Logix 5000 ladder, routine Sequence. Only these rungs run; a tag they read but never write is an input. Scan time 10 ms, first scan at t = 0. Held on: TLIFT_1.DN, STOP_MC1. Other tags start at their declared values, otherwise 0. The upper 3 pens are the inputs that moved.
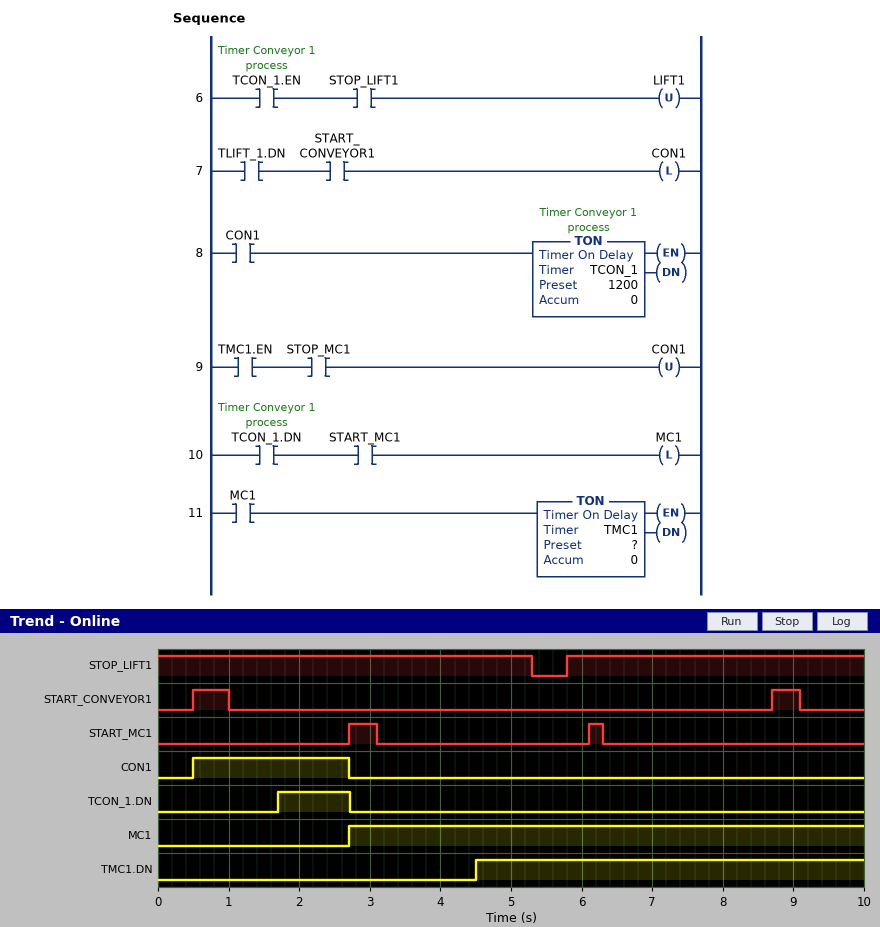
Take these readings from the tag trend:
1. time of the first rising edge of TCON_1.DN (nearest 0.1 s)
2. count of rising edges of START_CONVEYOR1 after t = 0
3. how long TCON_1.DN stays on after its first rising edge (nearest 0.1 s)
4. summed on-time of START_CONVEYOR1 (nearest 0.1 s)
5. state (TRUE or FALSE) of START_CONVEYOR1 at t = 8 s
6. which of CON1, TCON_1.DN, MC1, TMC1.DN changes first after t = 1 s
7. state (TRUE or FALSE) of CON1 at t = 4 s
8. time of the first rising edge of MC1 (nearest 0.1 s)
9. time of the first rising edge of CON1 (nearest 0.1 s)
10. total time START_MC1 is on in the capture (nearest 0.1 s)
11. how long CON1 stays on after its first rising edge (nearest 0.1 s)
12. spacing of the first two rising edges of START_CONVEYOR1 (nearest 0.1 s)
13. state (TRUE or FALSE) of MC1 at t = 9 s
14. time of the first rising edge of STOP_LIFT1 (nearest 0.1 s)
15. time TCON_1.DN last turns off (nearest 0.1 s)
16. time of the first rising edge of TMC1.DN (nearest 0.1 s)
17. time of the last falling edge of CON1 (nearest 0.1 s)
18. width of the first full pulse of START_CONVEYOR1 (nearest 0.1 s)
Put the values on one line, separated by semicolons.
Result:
1.7 s; 2; 1.0 s; 0.9 s; FALSE; TCON_1.DN; FALSE; 2.7 s; 0.5 s; 0.6 s; 2.2 s; 8.2 s; TRUE; 5.8 s; 2.7 s; 4.5 s; 2.7 s; 0.5 s
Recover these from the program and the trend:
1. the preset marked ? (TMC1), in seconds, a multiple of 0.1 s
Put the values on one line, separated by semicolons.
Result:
1.8 s
